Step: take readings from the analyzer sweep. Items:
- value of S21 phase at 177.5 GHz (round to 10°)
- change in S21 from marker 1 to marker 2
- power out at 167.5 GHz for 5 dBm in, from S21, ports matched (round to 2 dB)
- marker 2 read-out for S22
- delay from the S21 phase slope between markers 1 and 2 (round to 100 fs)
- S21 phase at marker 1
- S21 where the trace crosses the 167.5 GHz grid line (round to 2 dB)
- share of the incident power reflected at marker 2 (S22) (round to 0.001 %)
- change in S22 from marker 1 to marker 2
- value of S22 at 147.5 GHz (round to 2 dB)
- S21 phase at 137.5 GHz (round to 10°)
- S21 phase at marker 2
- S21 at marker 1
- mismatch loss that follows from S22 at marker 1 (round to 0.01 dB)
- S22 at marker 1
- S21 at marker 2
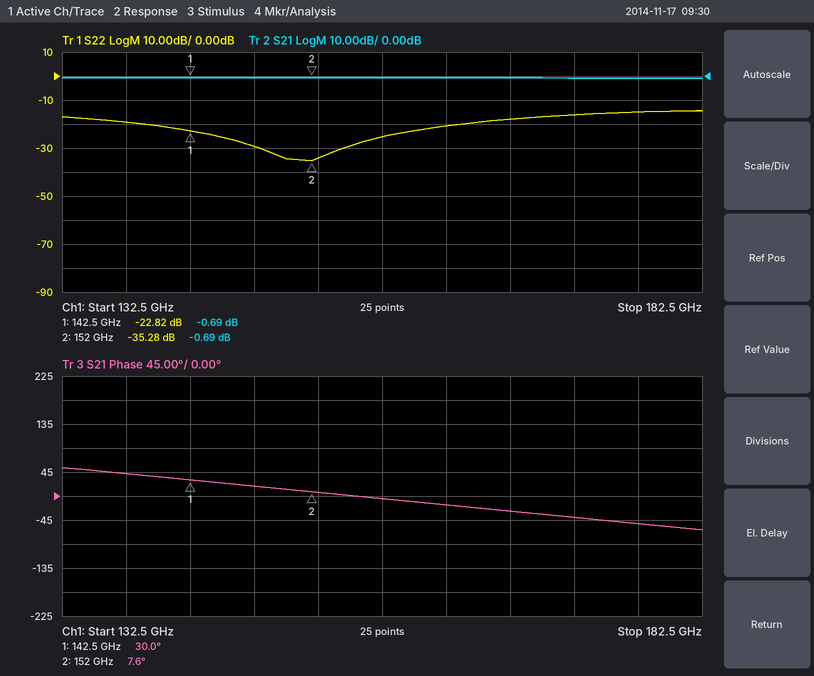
-50°
0.00 dB
4 dBm
-35.28 dB
6.5 ps
30.0°
0 dB
0.030 %
-12.46 dB
-30 dB
40°
7.6°
-0.69 dB
0.02 dB
-22.82 dB
-0.69 dB
